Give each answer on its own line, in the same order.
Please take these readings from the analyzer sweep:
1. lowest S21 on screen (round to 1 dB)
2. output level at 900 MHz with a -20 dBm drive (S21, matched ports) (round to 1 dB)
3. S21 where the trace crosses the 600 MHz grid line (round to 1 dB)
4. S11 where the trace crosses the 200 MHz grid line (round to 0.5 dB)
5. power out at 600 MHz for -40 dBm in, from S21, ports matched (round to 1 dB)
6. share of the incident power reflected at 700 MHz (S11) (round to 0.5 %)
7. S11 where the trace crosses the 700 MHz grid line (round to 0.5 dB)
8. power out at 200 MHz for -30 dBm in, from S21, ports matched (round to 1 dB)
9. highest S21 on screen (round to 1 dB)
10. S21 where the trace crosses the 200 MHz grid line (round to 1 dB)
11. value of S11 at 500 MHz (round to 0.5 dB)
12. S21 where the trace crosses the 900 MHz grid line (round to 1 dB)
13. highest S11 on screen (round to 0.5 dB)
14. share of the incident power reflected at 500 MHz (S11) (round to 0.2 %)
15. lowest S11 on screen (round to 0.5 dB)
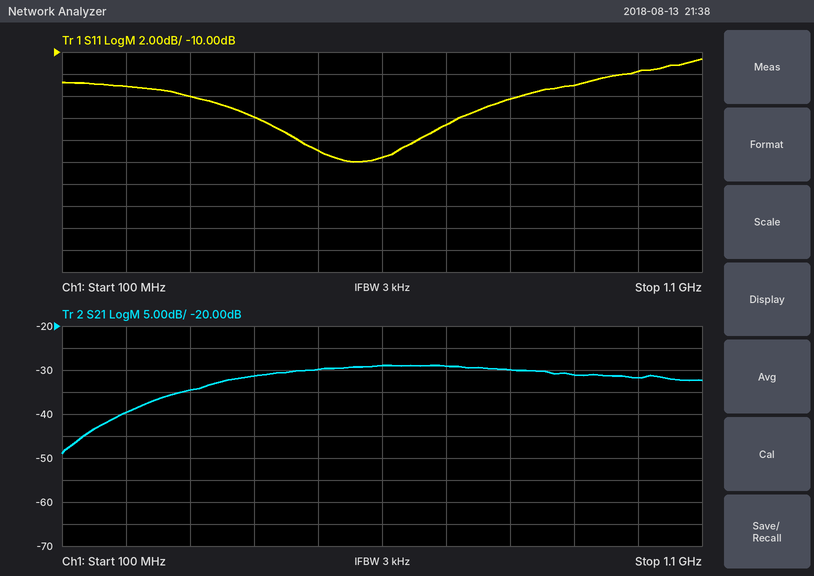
-49 dB
-51 dBm
-29 dB
-13.0 dB
-69 dBm
2.0 %
-16.5 dB
-70 dBm
-29 dB
-40 dB
-19.0 dB
-31 dB
-10.5 dB
1.2 %
-20.0 dB
